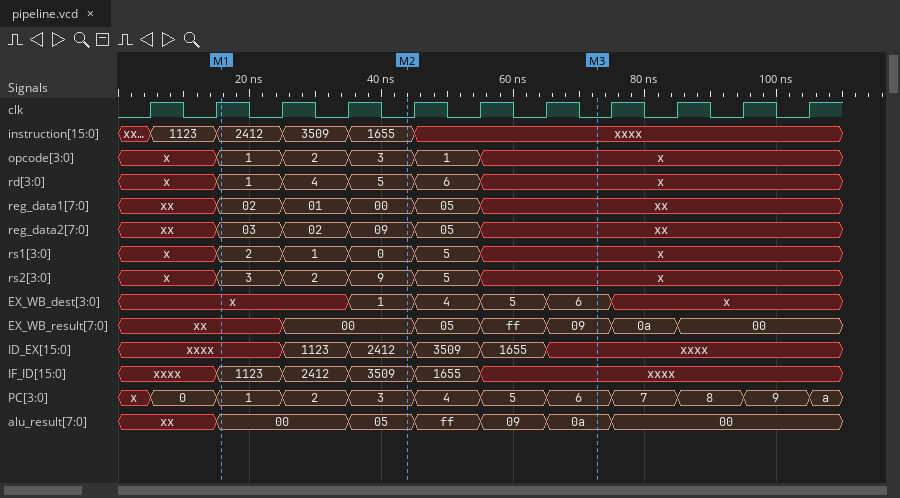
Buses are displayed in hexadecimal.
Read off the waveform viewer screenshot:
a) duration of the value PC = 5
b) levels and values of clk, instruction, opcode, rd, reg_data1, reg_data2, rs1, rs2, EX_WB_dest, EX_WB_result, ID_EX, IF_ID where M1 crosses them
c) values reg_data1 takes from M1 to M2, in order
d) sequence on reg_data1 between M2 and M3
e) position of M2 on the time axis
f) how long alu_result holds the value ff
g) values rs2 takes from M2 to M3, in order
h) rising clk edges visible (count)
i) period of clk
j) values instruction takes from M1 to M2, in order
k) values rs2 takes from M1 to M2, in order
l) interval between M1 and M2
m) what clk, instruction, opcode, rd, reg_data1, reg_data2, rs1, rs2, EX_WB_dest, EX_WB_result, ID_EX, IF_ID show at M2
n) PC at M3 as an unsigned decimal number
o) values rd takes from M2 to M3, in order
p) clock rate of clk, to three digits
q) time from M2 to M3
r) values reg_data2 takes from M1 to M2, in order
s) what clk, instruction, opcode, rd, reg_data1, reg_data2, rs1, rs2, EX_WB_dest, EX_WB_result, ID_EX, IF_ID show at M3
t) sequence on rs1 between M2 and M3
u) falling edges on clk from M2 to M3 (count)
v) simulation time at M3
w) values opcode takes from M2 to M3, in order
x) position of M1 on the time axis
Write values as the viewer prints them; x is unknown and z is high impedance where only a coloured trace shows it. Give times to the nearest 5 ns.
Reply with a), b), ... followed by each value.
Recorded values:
a) 10 ns
b) clk=1, instruction=2412, opcode=1, rd=1, reg_data1=02, reg_data2=03, rs1=2, rs2=3, EX_WB_dest=x, EX_WB_result=xx, ID_EX=xxxx, IF_ID=1123
c) 02, 01, 00
d) 00, 05, xx
e) 45 ns
f) 10 ns
g) 9, 5, x
h) 11
i) 10 ns
j) 2412, 3509, 1655
k) 3, 2, 9
l) 30 ns
m) clk=0, instruction=1655, opcode=3, rd=5, reg_data1=00, reg_data2=09, rs1=0, rs2=9, EX_WB_dest=1, EX_WB_result=00, ID_EX=2412, IF_ID=3509
n) 6
o) 5, 6, x
p) 100 MHz
q) 30 ns
r) 03, 02, 09
s) clk=0, instruction=xxxx, opcode=x, rd=x, reg_data1=xx, reg_data2=xx, rs1=x, rs2=x, EX_WB_dest=6, EX_WB_result=09, ID_EX=xxxx, IF_ID=xxxx
t) 0, 5, x
u) 3
v) 75 ns
w) 3, 1, x
x) 15 ns
